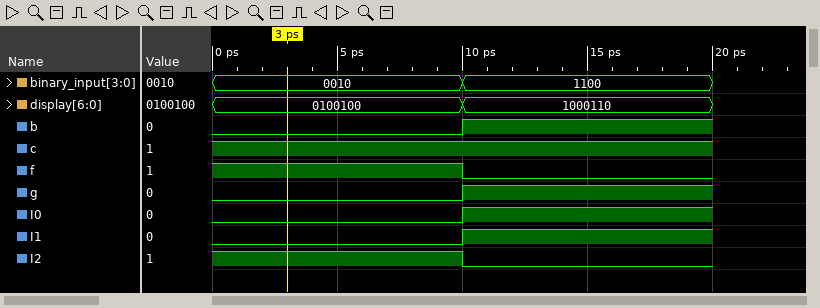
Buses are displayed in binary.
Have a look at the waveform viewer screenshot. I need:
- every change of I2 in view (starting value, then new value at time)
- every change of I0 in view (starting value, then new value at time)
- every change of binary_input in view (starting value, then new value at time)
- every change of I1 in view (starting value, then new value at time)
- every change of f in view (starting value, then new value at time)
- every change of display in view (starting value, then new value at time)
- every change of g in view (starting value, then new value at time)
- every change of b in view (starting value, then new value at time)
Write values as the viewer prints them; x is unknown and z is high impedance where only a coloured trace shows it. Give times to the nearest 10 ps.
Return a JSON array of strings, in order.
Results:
["1, 0 at 10 ps", "0, 1 at 10 ps", "0010, 1100 at 10 ps", "0, 1 at 10 ps", "1, 0 at 10 ps", "0100100, 1000110 at 10 ps", "0, 1 at 10 ps", "0, 1 at 10 ps"]
